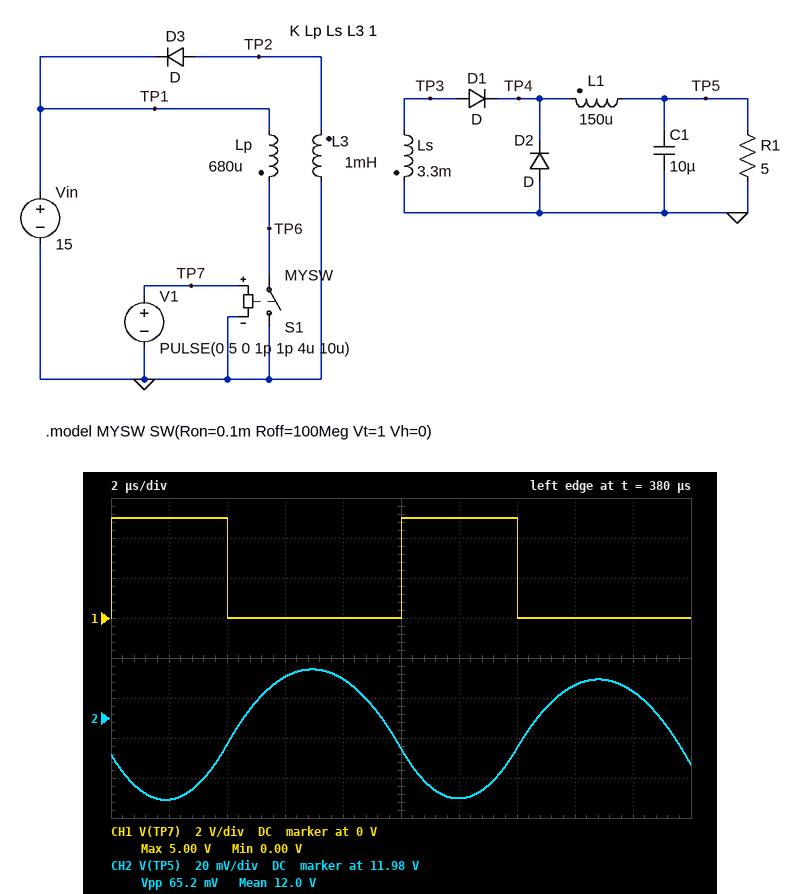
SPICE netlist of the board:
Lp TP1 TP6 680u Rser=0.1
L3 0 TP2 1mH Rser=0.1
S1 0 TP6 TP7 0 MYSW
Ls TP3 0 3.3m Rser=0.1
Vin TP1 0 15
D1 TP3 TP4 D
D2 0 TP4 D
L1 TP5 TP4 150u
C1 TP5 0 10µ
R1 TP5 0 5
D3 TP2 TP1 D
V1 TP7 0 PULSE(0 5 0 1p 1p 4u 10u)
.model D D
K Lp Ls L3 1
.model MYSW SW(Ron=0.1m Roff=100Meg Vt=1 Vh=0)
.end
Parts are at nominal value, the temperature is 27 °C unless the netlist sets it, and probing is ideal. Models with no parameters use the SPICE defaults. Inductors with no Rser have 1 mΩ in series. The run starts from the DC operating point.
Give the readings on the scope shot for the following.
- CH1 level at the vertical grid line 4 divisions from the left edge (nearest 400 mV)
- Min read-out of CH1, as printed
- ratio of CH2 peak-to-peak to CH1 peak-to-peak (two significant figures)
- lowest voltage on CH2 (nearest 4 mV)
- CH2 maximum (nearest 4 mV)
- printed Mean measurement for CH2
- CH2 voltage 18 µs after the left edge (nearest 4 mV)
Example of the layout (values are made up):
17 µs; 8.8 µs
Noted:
0 V; 0.00 V; 0.013; 11.940 V; 12.004 V; 12.0 V; 11.992 V
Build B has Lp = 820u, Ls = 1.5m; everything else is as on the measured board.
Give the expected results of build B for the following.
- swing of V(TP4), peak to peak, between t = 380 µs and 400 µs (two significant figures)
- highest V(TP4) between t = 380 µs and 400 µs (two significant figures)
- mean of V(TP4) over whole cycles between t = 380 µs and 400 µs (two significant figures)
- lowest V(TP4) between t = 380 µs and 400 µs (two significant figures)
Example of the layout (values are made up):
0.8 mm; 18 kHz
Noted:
20 V; 19 V; 7.1 V; -850 mV
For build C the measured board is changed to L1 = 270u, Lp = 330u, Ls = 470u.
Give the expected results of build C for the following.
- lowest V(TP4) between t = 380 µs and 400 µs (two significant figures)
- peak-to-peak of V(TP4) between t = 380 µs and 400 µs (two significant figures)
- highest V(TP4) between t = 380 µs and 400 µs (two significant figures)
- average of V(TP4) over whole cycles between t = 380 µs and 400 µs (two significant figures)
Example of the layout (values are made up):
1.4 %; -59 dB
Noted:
-840 mV; 18 V; 17 V; 6.2 V
